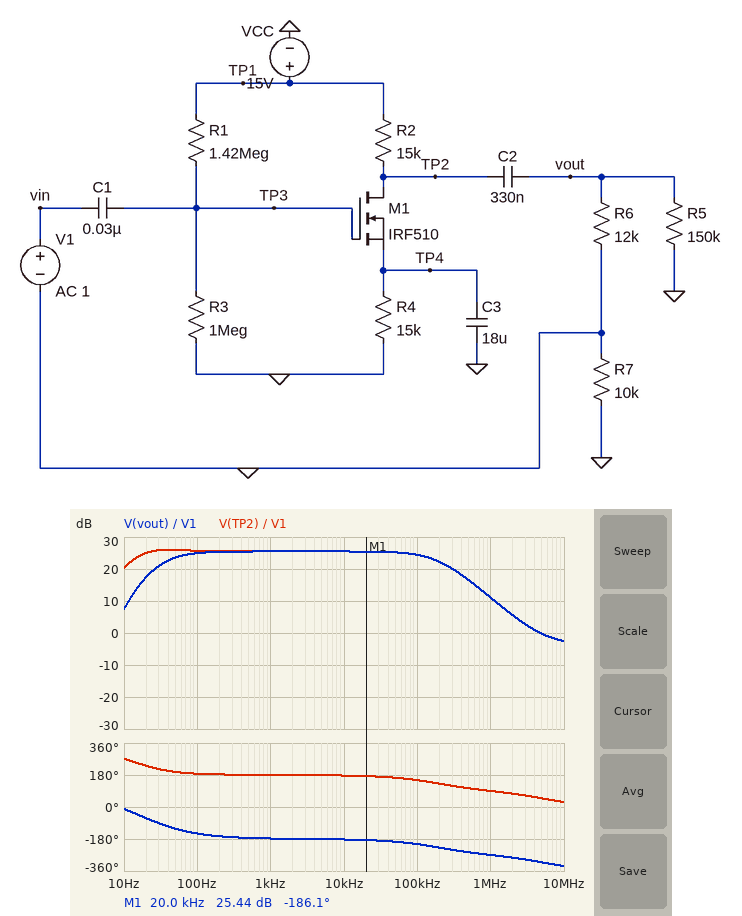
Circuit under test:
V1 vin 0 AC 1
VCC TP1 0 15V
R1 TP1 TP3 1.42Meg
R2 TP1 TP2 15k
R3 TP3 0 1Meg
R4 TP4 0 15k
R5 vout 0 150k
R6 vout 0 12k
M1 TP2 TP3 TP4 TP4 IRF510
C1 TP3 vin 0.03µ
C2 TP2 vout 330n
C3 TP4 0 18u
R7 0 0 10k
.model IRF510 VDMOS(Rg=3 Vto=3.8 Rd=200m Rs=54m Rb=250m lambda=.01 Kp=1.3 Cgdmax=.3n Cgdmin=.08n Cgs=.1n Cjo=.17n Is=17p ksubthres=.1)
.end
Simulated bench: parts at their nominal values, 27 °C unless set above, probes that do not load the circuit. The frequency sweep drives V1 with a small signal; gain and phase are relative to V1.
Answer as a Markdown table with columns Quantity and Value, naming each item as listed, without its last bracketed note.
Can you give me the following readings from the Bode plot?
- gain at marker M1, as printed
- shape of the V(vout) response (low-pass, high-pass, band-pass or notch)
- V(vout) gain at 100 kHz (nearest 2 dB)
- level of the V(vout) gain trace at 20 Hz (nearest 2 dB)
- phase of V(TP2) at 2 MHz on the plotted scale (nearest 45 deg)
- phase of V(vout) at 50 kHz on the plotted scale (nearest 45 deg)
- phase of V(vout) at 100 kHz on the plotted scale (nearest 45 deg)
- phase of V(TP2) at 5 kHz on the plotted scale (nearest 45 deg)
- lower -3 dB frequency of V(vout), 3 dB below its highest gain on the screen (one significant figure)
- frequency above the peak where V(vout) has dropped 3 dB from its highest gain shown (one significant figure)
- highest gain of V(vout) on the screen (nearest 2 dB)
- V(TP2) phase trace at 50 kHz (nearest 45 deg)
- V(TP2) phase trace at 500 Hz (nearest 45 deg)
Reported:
| Quantity | Value |
|---|---|
| gain at marker M1, as printed | 25.44 dB |
| shape of the V(vout) response | band-pass |
| V(vout) gain at 100 kHz | 24 dB |
| level of the V(vout) gain trace at 20 Hz | 18 dB |
| phase of V(TP2) at 2 MHz on the plotted scale | 90 deg |
| phase of V(vout) at 50 kHz on the plotted scale | -180 deg |
| phase of V(vout) at 100 kHz on the plotted scale | -225 deg |
| phase of V(TP2) at 5 kHz on the plotted scale | 180 deg |
| lower -3 dB frequency of V(vout), 3 dB below its highest gain on the screen | 40 Hz |
| frequency above the peak where V(vout) has dropped 3 dB from its highest gain shown | 200 kHz |
| highest gain of V(vout) on the screen | 26 dB |
| V(TP2) phase trace at 50 kHz | 180 deg |
| V(TP2) phase trace at 500 Hz | 180 deg |
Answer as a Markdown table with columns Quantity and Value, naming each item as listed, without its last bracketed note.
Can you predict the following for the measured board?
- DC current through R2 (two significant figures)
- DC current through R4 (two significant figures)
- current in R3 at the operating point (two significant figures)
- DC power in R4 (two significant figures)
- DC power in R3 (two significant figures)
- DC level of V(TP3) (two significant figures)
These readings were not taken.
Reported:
| Quantity | Value |
|---|---|
| DC current through R2 | 170 µA |
| DC current through R4 | 170 µA |
| current in R3 at the operating point | 6.2 µA |
| DC power in R4 | 440 µW |
| DC power in R3 | 38 µW |
| DC level of V(TP3) | 6.2 V |
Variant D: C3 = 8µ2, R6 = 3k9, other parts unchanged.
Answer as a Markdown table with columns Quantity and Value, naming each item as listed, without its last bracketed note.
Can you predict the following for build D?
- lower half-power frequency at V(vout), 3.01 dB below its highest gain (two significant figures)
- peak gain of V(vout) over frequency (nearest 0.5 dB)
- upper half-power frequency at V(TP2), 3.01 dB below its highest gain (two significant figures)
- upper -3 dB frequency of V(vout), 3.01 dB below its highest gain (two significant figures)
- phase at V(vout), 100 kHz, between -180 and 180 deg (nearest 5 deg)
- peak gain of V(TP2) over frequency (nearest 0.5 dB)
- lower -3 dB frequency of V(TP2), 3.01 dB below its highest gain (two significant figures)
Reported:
| Quantity | Value |
|---|---|
| lower half-power frequency at V(vout), 3.01 dB below its highest gain | 74 Hz |
| peak gain of V(vout) over frequency | 19.5 dB |
| upper half-power frequency at V(TP2), 3.01 dB below its highest gain | 370 Hz |
| upper -3 dB frequency of V(vout), 3.01 dB below its highest gain | 390 kHz |
| phase at V(vout), 100 kHz, between -180 and 180 deg | 165 deg |
| peak gain of V(TP2) over frequency | 22.5 dB |
| lower -3 dB frequency of V(TP2), 3.01 dB below its highest gain | 18 Hz |
